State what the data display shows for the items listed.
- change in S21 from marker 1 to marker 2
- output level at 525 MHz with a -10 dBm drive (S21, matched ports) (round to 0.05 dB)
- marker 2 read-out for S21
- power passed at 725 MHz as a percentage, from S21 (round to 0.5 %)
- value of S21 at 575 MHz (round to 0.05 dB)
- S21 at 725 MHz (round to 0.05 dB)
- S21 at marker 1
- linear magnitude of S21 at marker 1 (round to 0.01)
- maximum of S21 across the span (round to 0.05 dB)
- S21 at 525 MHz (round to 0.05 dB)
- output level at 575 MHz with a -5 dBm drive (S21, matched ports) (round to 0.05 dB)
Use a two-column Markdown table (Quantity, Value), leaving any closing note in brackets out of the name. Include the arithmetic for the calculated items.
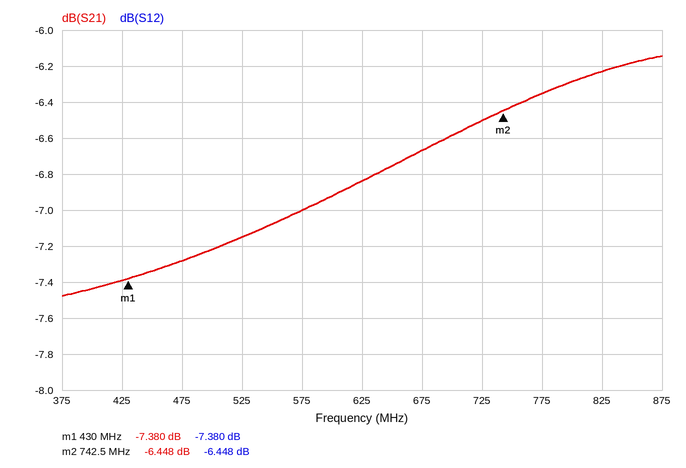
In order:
| Quantity | Value |
|---|---|
| change in S21 from marker 1 to marker 2 | -6.448 − (-7.38) = 0.932 dB |
| output level at 525 MHz with a -10 dBm drive (S21, matched ports) | -10 dBm + (-7.15 dB) = -17.15 dBm |
| marker 2 read-out for S21 | -6.448 dB |
| power passed at 725 MHz as a percentage, from S21 | 10^(-6.5/10) ≈ 22.4 %, so 22.5 % to the nearest 0.5 % |
| value of S21 at 575 MHz | -7.00 dB |
| S21 at 725 MHz | -6.50 dB |
| S21 at marker 1 | -7.380 dB |
| linear magnitude of S21 at marker 1 | 10^(-7.38/20) ≈ 0.43 |
| maximum of S21 across the span | -6.15 dB |
| S21 at 525 MHz | -7.15 dB |
| output level at 575 MHz with a -5 dBm drive (S21, matched ports) | -5 dBm + (-7.00 dB) = -12.00 dBm |
